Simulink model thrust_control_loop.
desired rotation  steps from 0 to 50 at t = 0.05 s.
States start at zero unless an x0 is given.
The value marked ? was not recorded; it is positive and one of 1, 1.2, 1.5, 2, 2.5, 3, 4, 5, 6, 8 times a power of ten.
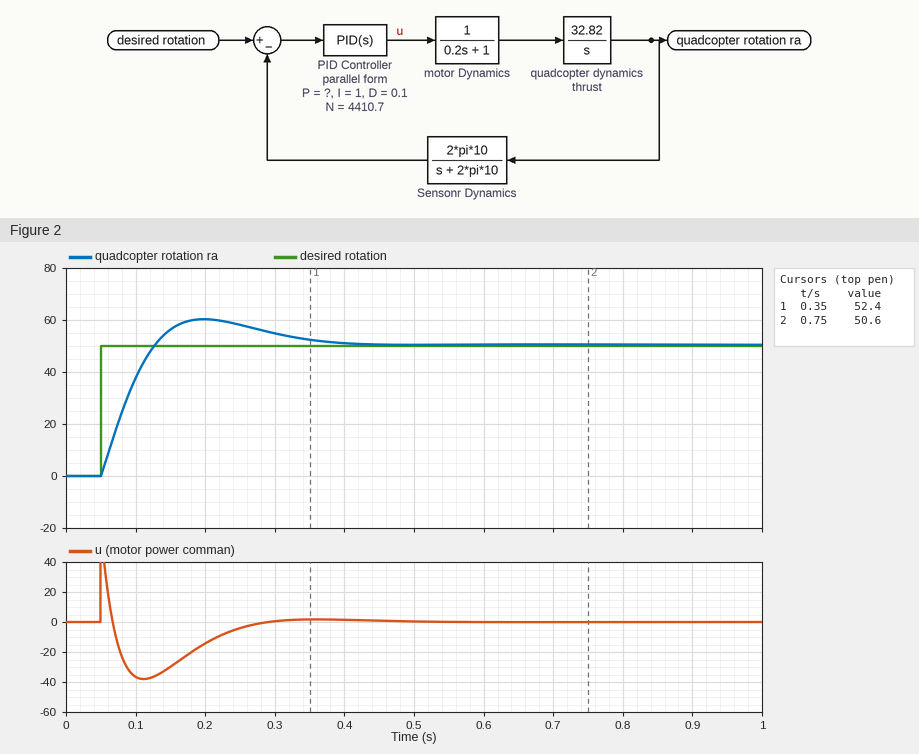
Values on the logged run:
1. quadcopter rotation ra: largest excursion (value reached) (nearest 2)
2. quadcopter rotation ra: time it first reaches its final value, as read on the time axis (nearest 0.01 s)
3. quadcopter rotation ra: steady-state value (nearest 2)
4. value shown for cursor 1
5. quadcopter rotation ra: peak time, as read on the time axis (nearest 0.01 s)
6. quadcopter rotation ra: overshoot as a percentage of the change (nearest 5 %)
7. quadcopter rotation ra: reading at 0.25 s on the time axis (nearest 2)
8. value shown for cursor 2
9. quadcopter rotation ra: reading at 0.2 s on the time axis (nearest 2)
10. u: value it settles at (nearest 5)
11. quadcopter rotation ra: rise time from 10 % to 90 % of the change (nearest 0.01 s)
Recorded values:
60
0.13 s
50
52.4
0.20 s
20 %
58
50.6
60
0
0.06 s
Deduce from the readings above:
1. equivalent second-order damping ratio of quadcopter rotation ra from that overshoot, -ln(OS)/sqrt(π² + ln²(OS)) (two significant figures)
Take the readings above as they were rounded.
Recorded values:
0.46
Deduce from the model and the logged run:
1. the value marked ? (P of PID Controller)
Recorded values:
1.2
